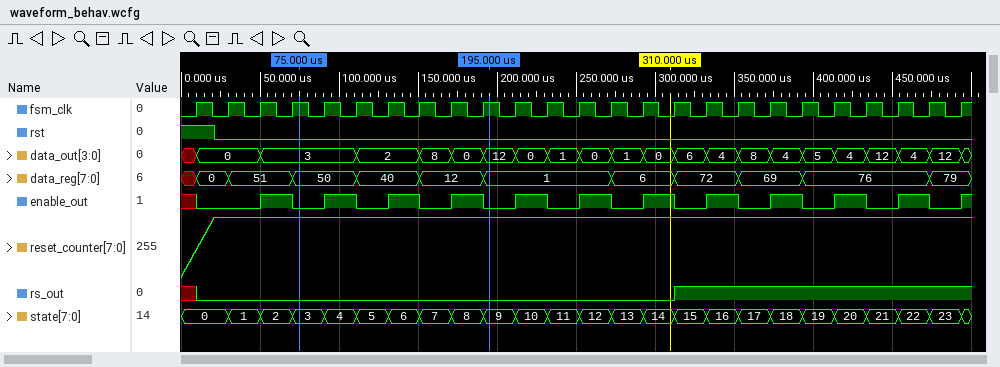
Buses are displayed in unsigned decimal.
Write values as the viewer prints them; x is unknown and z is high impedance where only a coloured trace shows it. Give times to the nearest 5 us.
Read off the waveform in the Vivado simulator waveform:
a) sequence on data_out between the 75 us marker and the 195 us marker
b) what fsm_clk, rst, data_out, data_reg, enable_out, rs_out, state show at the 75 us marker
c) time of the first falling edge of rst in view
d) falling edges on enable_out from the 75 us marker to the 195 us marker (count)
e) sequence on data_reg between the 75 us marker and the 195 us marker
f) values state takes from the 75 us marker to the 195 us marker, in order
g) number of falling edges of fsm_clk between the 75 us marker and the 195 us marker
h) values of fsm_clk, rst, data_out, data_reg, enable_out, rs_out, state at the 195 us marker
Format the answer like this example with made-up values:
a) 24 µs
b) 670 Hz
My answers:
a) 3, 2, 8, 0, 12
b) fsm_clk=1, rst=0, data_out=3, data_reg=50, enable_out=0, rs_out=0, state=3
c) 20 us
d) 3
e) 50, 40, 12, 1
f) 3, 4, 5, 6, 7, 8, 9
g) 6
h) fsm_clk=1, rst=0, data_out=12, data_reg=1, enable_out=0, rs_out=0, state=9
